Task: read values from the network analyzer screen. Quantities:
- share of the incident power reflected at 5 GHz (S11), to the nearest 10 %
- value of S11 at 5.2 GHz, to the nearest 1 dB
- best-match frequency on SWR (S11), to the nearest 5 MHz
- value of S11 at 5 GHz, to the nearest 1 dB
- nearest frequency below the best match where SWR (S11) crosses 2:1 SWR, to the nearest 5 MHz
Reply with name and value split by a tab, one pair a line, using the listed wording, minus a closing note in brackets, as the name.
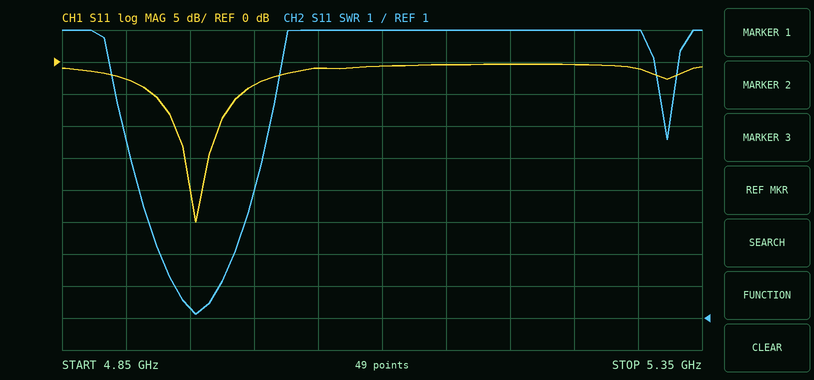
share of the incident power reflected at 5 GHz (S11), to the nearest 10 %	40 %
value of S11 at 5.2 GHz, to the nearest 1 dB	0 dB
best-match frequency on SWR (S11), to the nearest 5 MHz	4.955 GHz
value of S11 at 5 GHz, to the nearest 1 dB	-4 dB
nearest frequency below the best match where SWR (S11) crosses 2:1 SWR, to the nearest 5 MHz	4.940 GHz
